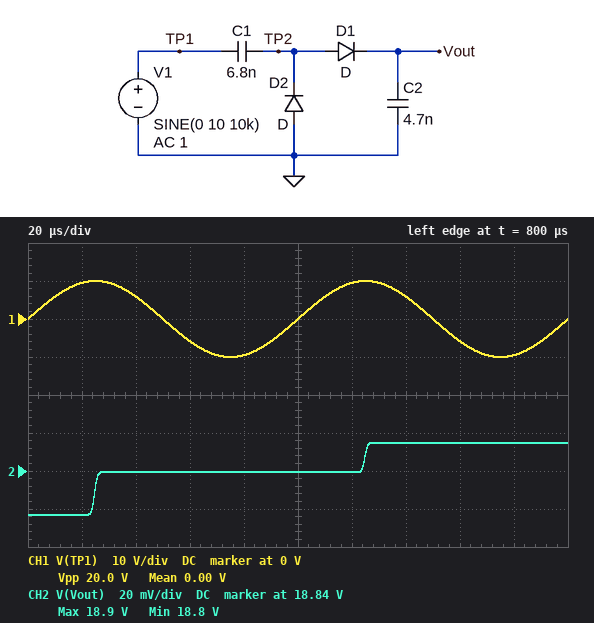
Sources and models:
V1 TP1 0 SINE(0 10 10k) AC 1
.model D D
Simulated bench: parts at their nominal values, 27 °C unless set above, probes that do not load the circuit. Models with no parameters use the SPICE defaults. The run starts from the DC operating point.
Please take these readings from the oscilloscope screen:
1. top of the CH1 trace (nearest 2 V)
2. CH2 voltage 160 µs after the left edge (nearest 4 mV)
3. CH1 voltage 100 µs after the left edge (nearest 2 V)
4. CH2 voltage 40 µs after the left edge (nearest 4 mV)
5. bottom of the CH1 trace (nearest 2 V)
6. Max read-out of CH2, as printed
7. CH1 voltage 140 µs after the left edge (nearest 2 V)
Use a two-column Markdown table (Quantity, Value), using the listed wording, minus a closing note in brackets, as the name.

| Quantity | Value |
|---|---|
| top of the CH1 trace | 10 V |
| CH2 voltage 160 µs after the left edge | 18.856 V |
| CH1 voltage 100 µs after the left edge | 0 V |
| CH2 voltage 40 µs after the left edge | 18.840 V |
| bottom of the CH1 trace | -10 V |
| Max read-out of CH2, as printed | 18.9 V |
| CH1 voltage 140 µs after the left edge | 6 V |
